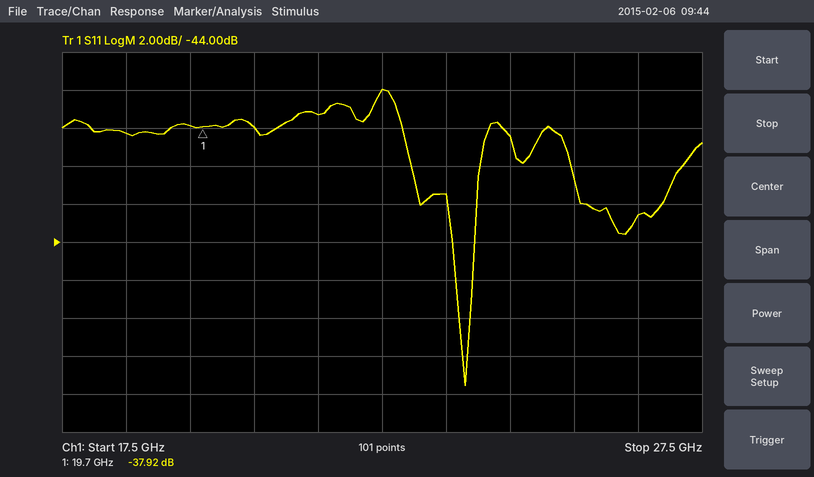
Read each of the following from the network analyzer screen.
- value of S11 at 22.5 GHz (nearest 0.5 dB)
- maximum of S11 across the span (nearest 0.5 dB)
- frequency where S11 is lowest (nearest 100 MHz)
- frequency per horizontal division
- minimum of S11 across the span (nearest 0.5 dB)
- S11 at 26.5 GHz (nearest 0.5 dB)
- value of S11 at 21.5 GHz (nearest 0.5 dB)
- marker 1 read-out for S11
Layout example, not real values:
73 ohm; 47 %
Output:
-36.0 dB; -36.0 dB; 23.8 GHz; 1 GHz; -51.5 dB; -42.5 dB; -37.5 dB; -37.92 dB
